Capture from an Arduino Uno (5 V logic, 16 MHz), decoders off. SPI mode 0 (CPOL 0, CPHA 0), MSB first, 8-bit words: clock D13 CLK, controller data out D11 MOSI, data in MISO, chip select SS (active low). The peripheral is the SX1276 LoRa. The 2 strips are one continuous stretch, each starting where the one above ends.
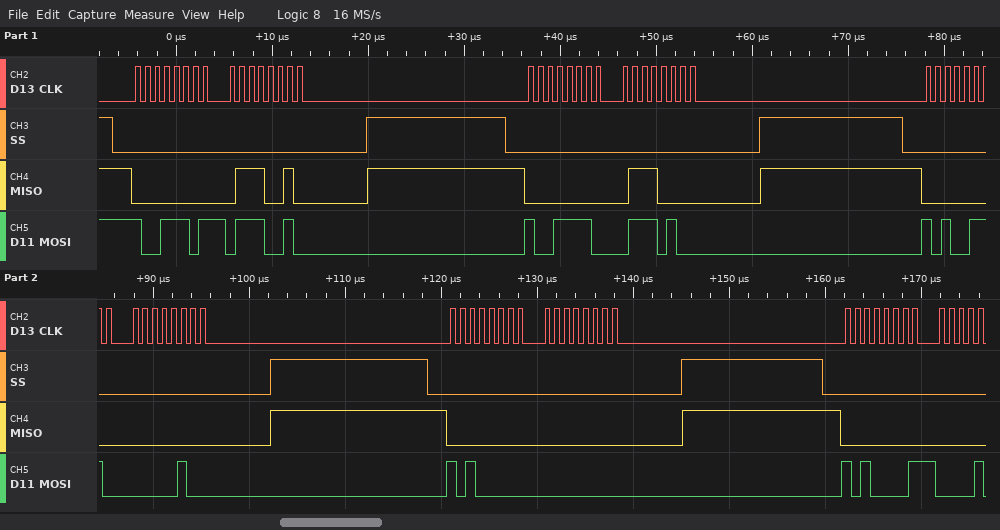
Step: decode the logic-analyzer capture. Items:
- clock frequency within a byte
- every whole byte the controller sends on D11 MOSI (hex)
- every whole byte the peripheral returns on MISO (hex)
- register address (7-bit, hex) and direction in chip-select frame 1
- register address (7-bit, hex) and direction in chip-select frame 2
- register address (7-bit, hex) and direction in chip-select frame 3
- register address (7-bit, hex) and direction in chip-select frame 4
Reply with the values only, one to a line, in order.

1 MHz
0x9D 0x72 0x9E 0x74 0xA6 0x04 0xA0 0x00 0xA1
0x00 0x72 0x00 0x70 0x00 0x00 0x00 0x00 0x00
0x1D write
0x1E write
0x26 write
0x20 write
